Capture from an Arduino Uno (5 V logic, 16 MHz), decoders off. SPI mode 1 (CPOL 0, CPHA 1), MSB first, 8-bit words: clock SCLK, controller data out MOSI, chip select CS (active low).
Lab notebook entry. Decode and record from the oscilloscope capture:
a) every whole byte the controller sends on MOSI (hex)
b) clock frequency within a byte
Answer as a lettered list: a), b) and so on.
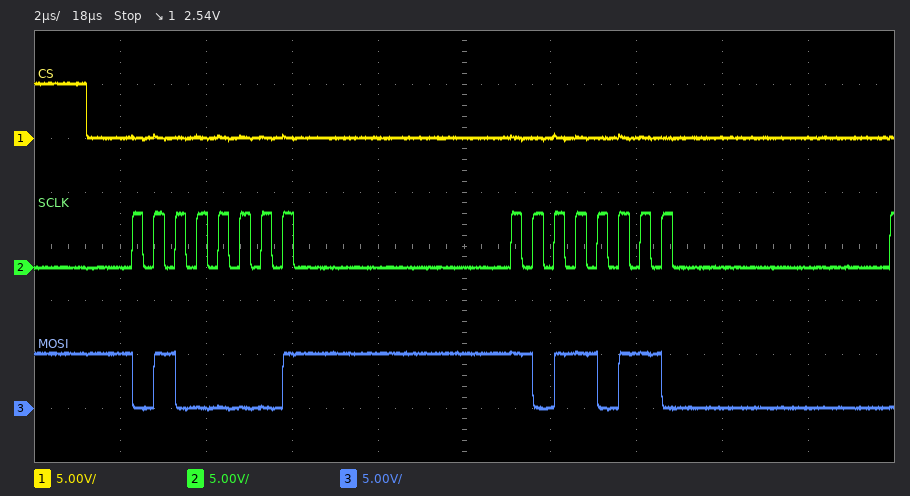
a) 0x41 0xB6
b) 2 MHz
